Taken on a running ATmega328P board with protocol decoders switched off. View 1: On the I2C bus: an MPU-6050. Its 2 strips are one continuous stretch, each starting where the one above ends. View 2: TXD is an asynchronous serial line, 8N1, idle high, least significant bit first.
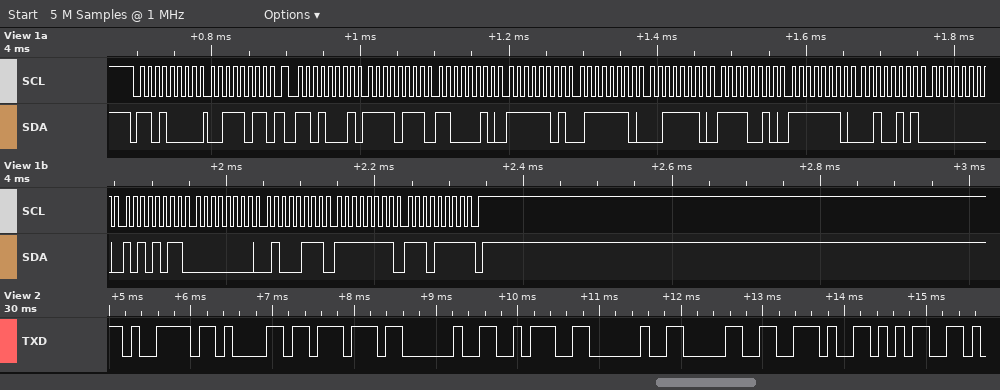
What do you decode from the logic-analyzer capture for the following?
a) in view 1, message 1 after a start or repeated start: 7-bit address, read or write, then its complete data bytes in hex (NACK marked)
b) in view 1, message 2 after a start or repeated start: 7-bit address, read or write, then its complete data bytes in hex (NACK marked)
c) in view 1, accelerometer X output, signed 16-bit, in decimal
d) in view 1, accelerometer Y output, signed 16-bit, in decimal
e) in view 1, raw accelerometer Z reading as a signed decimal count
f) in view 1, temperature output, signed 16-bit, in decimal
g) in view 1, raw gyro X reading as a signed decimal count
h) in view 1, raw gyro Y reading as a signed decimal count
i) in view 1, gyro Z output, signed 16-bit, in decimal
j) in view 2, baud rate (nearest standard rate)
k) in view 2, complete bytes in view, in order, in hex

0x68 write: 3B
0x68 read: F7 C2 FD 7E 3E F2 FE 25 00 AB 00 47 FF EF NACK
-2110
-642
16114
-475
171
71
-17
9600 baud
79 61 77 20 3A 20 30 2E 35
